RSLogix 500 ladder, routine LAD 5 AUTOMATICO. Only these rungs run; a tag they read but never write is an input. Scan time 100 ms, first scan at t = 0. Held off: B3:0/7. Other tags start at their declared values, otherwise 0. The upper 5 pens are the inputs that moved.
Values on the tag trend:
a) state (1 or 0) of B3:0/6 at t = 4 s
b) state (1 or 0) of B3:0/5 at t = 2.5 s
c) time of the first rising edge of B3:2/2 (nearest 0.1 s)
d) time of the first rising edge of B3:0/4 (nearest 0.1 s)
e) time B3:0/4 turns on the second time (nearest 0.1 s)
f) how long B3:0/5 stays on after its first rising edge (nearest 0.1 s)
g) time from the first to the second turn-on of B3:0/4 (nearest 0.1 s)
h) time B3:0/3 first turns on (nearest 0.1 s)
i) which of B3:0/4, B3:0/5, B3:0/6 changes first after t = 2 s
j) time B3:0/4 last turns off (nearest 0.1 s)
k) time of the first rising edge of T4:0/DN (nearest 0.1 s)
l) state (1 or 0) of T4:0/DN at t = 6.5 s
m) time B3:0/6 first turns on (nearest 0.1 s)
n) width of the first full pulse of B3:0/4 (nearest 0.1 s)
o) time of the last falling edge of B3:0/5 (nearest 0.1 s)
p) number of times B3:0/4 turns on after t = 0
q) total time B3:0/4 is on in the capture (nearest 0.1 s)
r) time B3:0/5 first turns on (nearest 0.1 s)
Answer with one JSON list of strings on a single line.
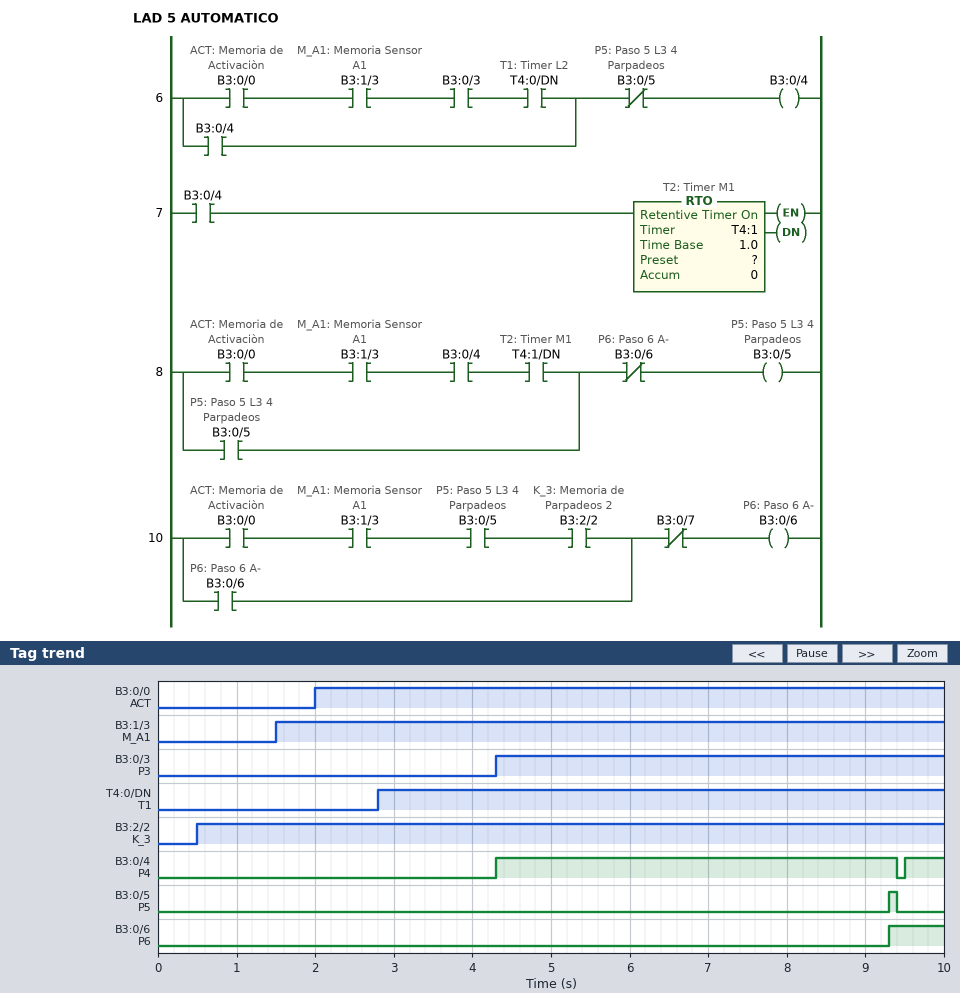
["0", "0", "0.5 s", "4.3 s", "9.5 s", "0.1 s", "5.2 s", "4.3 s", "B3:0/4", "9.4 s", "2.8 s", "1", "9.3 s", "5.1 s", "9.4 s", "2", "5.6 s", "9.3 s"]
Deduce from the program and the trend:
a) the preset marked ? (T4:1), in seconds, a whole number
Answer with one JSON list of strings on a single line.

["5 s"]
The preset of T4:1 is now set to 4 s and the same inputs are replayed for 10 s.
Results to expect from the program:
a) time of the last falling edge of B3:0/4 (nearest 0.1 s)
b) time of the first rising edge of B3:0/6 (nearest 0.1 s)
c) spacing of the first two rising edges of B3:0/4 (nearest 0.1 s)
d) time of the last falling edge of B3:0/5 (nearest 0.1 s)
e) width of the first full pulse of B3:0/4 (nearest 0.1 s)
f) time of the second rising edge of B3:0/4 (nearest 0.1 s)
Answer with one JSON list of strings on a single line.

["8.4 s", "8.3 s", "4.2 s", "8.4 s", "4.1 s", "8.5 s"]
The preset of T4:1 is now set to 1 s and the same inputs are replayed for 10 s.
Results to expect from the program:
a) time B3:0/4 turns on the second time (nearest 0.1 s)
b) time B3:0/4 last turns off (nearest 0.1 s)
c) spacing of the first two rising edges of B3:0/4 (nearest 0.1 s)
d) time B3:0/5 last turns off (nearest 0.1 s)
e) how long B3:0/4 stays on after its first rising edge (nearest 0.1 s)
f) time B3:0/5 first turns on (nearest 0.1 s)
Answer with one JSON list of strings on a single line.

["5.5 s", "5.4 s", "1.2 s", "5.4 s", "1.1 s", "5.3 s"]
